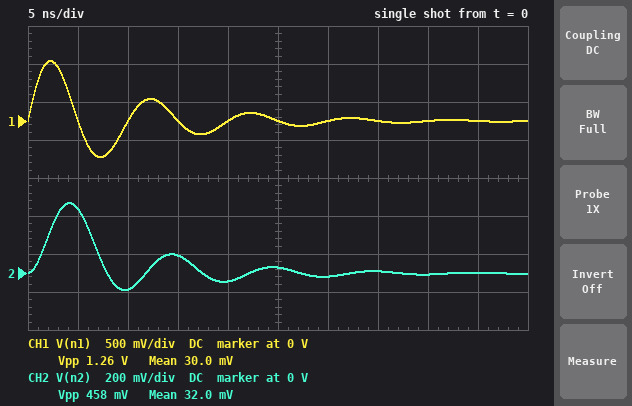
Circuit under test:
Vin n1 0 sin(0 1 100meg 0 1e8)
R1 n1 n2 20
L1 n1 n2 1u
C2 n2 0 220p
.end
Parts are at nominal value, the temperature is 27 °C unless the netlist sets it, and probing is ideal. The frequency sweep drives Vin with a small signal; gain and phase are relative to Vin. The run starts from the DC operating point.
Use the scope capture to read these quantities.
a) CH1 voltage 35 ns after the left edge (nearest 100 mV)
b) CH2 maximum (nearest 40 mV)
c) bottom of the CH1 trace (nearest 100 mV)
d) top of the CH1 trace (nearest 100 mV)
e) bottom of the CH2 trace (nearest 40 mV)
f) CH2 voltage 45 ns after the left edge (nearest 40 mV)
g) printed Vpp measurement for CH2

0 V
360 mV
-500 mV
800 mV
-80 mV
0 V
458 mV
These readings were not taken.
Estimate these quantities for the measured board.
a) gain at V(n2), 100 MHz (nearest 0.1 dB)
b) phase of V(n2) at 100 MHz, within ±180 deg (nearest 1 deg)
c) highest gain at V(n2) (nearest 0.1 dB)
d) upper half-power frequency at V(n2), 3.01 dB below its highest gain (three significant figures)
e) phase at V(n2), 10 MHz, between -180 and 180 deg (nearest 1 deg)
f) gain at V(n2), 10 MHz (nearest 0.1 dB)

-9.3 dB
-72 deg
0.5 dB
35.3 MHz
-15 deg
0.4 dB
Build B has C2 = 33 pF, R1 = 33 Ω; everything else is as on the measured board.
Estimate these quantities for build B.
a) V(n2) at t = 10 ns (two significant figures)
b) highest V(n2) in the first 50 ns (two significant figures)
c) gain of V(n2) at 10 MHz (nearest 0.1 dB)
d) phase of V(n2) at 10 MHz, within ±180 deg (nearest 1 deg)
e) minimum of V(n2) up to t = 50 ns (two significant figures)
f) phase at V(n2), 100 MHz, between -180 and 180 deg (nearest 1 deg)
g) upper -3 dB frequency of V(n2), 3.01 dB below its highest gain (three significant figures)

-210 mV
680 mV
0.2 dB
-3 deg
-390 mV
-35 deg
143 MHz
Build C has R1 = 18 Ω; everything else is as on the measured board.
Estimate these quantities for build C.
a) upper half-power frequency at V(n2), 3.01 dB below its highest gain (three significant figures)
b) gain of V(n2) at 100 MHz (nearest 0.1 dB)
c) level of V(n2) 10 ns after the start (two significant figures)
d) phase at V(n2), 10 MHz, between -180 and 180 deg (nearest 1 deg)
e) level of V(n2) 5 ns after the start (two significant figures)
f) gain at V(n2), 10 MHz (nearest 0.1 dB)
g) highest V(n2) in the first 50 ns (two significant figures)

39.2 MHz
-8.5 dB
-110 mV
-14 deg
350 mV
0.3 dB
390 mV
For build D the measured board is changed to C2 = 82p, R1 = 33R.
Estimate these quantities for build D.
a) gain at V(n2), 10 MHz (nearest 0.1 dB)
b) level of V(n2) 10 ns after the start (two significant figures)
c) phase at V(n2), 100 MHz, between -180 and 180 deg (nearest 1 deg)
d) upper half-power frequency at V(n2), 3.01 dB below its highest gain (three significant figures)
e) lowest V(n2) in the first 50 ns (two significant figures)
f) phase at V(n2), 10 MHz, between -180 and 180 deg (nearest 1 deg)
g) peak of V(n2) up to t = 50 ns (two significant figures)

0.5 dB
-180 mV
-62 deg
57.3 MHz
-200 mV
-8 deg
490 mV
